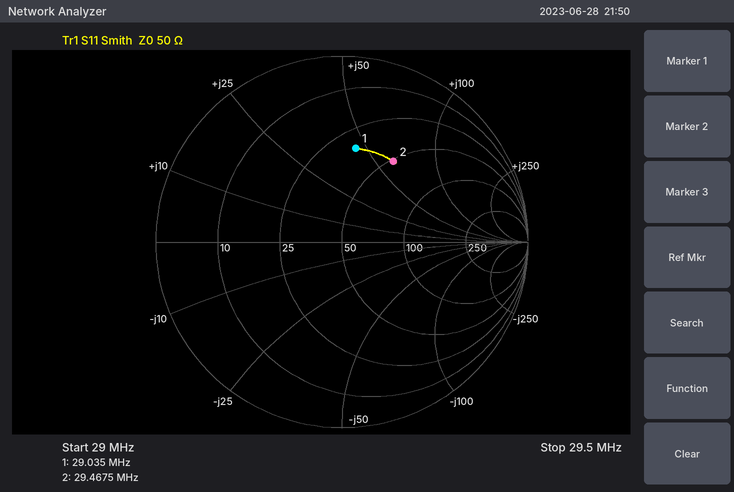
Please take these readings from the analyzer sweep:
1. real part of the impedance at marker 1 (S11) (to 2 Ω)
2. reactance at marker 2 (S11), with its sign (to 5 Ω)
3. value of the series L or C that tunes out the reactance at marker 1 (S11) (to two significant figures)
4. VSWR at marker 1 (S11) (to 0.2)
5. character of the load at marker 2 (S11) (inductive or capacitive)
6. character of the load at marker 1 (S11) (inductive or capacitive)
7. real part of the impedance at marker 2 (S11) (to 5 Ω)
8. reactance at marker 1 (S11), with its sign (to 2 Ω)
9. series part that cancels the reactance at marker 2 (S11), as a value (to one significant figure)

34 Ω
+60 Ω
120 pF
3.0
inductive
inductive
50 Ω
+46 Ω
90 pF
